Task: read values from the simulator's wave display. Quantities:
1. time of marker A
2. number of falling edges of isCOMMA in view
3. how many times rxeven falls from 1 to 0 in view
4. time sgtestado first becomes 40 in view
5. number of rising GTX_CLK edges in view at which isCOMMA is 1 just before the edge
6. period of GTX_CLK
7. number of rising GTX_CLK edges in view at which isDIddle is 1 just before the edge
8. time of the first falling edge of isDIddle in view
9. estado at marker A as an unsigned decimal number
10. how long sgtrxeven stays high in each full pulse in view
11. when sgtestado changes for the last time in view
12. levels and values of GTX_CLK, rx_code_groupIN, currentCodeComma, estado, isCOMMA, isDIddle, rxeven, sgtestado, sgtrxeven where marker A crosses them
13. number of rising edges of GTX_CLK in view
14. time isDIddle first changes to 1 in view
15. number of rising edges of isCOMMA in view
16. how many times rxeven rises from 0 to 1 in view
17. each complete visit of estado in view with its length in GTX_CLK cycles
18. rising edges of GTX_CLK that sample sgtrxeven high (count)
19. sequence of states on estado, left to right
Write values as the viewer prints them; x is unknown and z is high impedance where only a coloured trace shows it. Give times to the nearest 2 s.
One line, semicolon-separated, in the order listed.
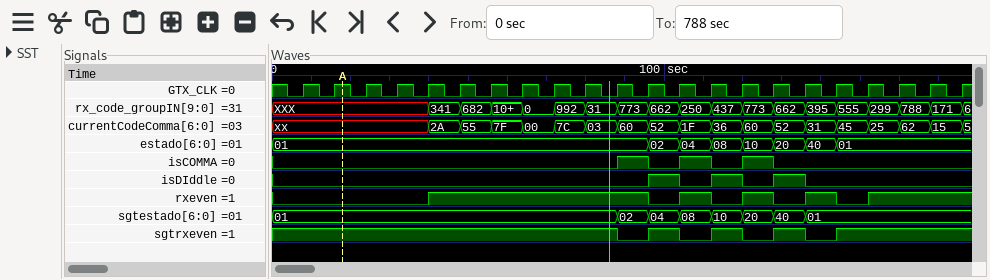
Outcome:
18 s; 3; 4; 128 s; 3; 8 s; 3; 104 s; 1; 8 s, 8 s, 8 s; 136 s; GTX_CLK=1, rx_code_groupIN=XXX, currentCodeComma=xx, estado=01, isCOMMA=0, isDIddle=0, rxeven=0, sgtestado=01, sgtrxeven=1; 22; 96 s; 3; 5; 02: 1, 04: 1, 08: 1, 10: 1, 20: 1, 40: 1; 18; 01, 02, 04, 08, 10, 20, 40, 01
